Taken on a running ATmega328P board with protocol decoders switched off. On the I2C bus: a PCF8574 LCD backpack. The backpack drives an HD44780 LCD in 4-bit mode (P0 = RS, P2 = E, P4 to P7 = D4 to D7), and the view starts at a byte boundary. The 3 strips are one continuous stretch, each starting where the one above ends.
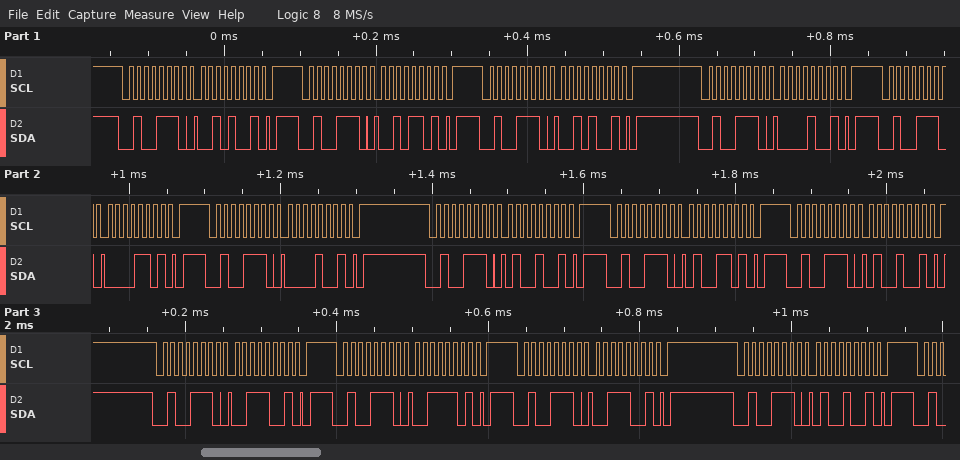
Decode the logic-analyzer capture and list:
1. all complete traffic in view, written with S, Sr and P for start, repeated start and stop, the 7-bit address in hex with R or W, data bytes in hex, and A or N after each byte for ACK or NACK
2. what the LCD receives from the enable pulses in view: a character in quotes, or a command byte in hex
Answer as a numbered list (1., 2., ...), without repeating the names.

1. S 27W A 29 A P S 27W A 2D A P S 27W A 29 A P S 27W A 09 A P S 27W A 0D A P S 27W A 09 A P S 27W A 49 A P S 27W A 4D A P S 27W A 49 A P S 27W A 39 A P S 27W A 3D A P S 27W A 39 A P S 27W A 49 A P
2. ' ' 'C'
